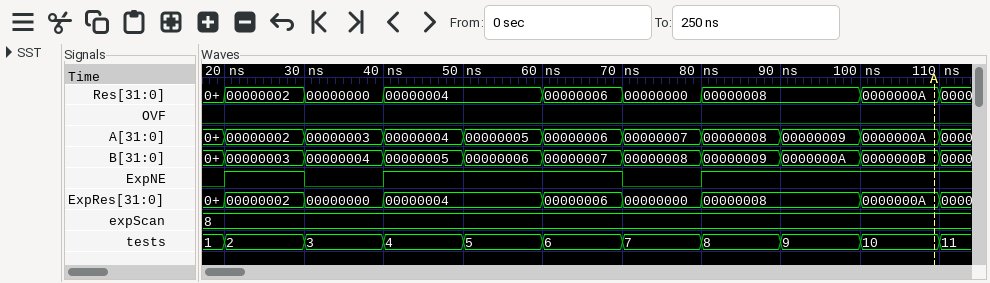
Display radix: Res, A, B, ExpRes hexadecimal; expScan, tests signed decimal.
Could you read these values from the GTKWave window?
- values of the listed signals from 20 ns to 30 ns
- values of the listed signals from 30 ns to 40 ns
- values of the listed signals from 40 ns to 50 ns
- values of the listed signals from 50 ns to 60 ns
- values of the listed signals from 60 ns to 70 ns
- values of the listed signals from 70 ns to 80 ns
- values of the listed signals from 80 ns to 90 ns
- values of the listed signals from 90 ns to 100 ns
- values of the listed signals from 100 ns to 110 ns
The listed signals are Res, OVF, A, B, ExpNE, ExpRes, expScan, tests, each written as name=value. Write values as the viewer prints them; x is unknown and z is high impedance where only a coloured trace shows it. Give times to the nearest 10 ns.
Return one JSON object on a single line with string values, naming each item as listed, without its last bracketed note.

{"values of the listed signals from 20 ns to 30 ns": "Res=00000002, OVF=0, A=00000002, B=00000003, ExpNE=1, ExpRes=00000002, expScan=8, tests=2", "values of the listed signals from 30 ns to 40 ns": "Res=00000000, OVF=0, A=00000003, B=00000004, ExpNE=0, ExpRes=00000000, expScan=8, tests=3", "values of the listed signals from 40 ns to 50 ns": "Res=00000004, OVF=0, A=00000004, B=00000005, ExpNE=1, ExpRes=00000004, expScan=8, tests=4", "values of the listed signals from 50 ns to 60 ns": "Res=00000004, OVF=0, A=00000005, B=00000006, ExpNE=1, ExpRes=00000004, expScan=8, tests=5", "values of the listed signals from 60 ns to 70 ns": "Res=00000006, OVF=0, A=00000006, B=00000007, ExpNE=1, ExpRes=00000006, expScan=8, tests=6", "values of the listed signals from 70 ns to 80 ns": "Res=00000000, OVF=0, A=00000007, B=00000008, ExpNE=0, ExpRes=00000000, expScan=8, tests=7", "values of the listed signals from 80 ns to 90 ns": "Res=00000008, OVF=0, A=00000008, B=00000009, ExpNE=1, ExpRes=00000008, expScan=8, tests=8", "values of the listed signals from 90 ns to 100 ns": "Res=00000008, OVF=0, A=00000009, B=0000000A, ExpNE=1, ExpRes=00000008, expScan=8, tests=9", "values of the listed signals from 100 ns to 110 ns": "Res=0000000A, OVF=0, A=0000000A, B=0000000B, ExpNE=1, ExpRes=0000000A, expScan=8, tests=10"}
